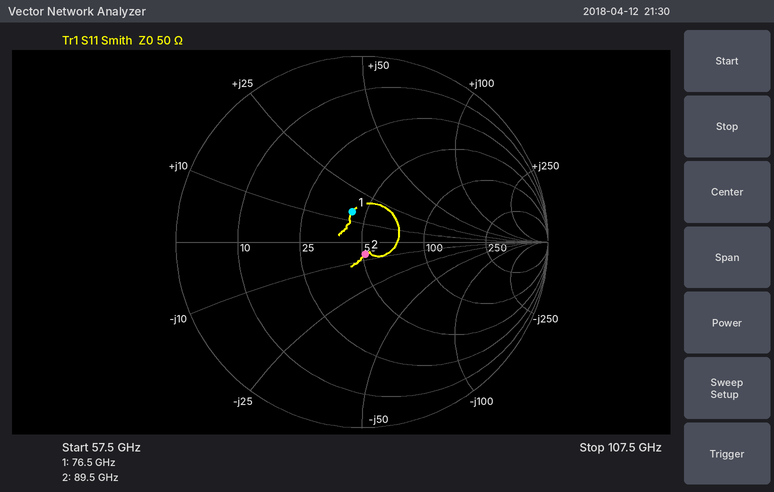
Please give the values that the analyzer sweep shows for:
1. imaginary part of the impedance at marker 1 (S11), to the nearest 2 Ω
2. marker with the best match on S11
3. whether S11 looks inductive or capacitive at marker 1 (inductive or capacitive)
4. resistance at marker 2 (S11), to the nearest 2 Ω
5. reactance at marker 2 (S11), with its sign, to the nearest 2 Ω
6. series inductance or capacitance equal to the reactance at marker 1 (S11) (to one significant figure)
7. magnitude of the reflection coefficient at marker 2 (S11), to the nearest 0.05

+14 Ω
marker 2
inductive
52 Ω
-6 Ω
30 pH
0.05
